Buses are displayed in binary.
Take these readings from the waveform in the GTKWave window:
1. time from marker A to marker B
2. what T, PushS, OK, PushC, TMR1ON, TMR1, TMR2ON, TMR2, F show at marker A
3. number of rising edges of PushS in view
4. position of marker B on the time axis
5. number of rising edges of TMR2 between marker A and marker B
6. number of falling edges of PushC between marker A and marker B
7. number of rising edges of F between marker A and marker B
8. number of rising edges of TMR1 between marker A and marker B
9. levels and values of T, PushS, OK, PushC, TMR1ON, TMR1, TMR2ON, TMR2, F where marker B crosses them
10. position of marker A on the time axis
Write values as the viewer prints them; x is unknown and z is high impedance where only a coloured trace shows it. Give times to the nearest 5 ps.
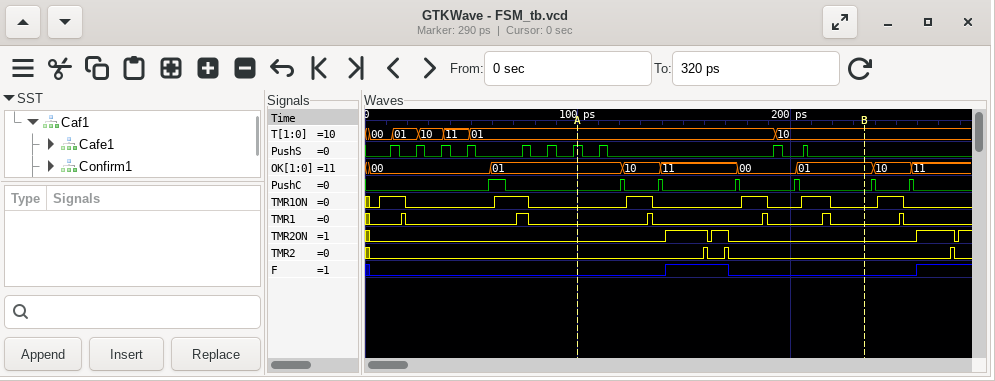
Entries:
135 ps
T=01, PushS=1, OK=01, PushC=0, TMR1ON=0, TMR1=0, TMR2ON=0, TMR2=0, F=0
10
235 ps
2
4
1
3
T=10, PushS=0, OK=01, PushC=0, TMR1ON=0, TMR1=0, TMR2ON=0, TMR2=0, F=0
100 ps
